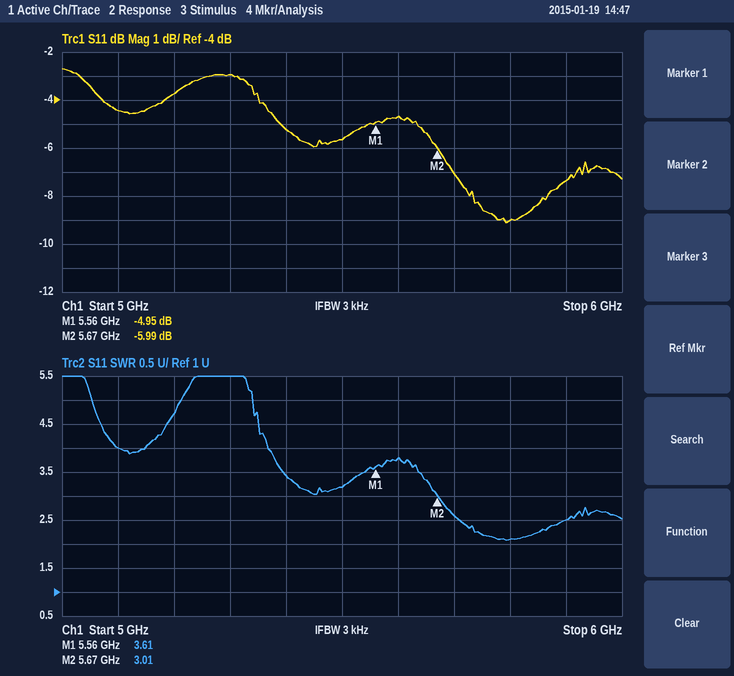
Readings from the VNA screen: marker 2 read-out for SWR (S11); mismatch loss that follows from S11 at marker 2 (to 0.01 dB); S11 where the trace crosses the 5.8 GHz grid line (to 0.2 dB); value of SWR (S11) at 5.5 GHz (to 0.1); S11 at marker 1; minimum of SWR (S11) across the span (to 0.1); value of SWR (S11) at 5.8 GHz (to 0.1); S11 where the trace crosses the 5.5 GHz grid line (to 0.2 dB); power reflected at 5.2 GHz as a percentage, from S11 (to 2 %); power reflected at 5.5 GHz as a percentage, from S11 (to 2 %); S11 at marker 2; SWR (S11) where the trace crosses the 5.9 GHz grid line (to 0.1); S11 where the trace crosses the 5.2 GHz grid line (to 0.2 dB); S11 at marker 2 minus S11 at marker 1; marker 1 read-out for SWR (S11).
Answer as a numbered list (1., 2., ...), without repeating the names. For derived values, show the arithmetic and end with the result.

1. 3.01
2. −10 log10(1 − 10^(-5.99/10)) ≈ 1.26 dB
3. -9.0 dB
4. 3.2
5. -4.95 dB
6. 2.1
7. 2.1
8. -5.6 dB
9. 10^(-3.8/10) ≈ 42 %
10. 10^(-5.6/10) ≈ 28 %
11. -5.99 dB
12. 2.5
13. -3.8 dB
14. -5.99 − (-4.95) = -1.04 dB
15. 3.61
